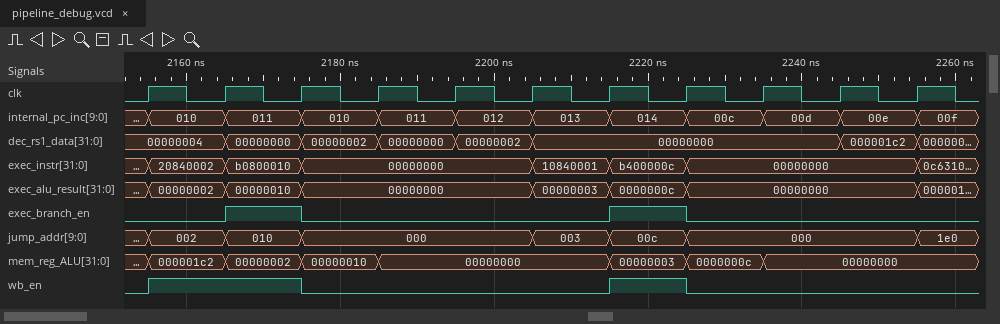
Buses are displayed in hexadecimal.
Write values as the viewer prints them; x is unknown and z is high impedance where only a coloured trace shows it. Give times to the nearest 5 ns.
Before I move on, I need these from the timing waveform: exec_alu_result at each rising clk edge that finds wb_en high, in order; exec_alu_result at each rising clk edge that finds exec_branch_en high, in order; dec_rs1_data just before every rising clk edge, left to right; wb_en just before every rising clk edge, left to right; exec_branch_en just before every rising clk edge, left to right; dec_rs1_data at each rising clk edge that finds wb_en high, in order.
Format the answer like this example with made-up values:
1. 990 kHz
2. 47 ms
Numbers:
1. 00000002, 00000010, 0000000c
2. 00000010, 0000000c
3. 00000004, 00000004, 00000000, 00000002, 00000000, 00000002, 00000000, 00000000, 00000000, 00000000, 000001c2
4. 0 1 1 0 0 0 0 1 0 0 0
5. 0 0 1 0 0 0 0 1 0 0 0
6. 00000004, 00000000, 00000000
